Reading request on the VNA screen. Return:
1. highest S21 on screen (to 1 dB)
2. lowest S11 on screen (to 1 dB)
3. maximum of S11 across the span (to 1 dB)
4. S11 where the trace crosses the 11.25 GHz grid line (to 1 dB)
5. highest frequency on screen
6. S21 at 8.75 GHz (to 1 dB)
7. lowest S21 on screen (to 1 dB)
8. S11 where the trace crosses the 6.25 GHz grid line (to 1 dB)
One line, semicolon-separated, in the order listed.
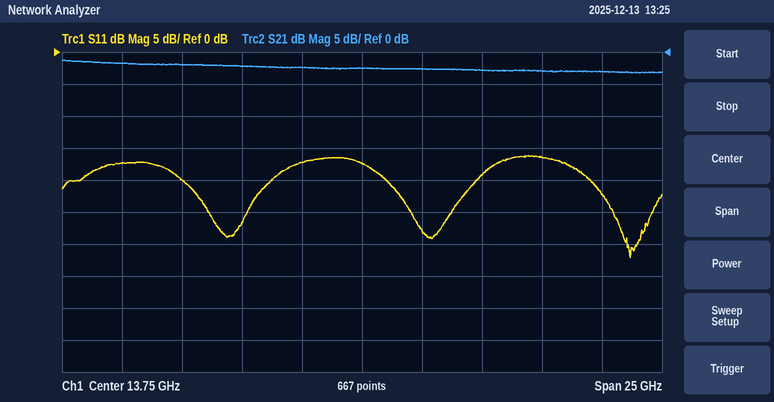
-1 dB; -32 dB; -16 dB; -17 dB; 26.25 GHz; -2 dB; -3 dB; -20 dB
